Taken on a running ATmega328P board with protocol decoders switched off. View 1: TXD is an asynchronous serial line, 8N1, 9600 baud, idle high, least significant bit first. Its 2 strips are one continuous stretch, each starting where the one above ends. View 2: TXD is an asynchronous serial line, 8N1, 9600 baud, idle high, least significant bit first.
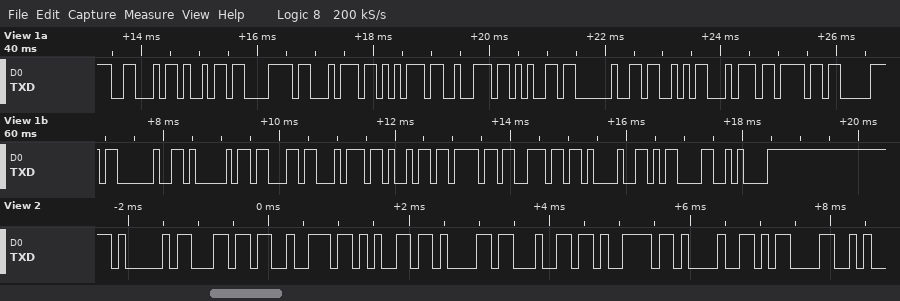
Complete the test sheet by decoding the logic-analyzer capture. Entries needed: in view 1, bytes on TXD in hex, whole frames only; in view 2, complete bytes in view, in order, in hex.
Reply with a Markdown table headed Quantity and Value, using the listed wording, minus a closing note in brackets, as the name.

| Quantity | Value |
|---|---|
| in view 1, bytes on TXD in hex, whole frames only | 0x46 0x69 0x78 0x74 0x75 0x72 0x65 0x20 0x53 0x74 0x6F 0x70 0x20 0x41 0x63 0x74 0x69 0x6F 0x6E 0x21 0x0D 0x0A |
| in view 2, complete bytes in view, in order, in hex | 0x41 0x6C 0x72 0x65 0x61 0x64 0x79 0x21 0x0D |
